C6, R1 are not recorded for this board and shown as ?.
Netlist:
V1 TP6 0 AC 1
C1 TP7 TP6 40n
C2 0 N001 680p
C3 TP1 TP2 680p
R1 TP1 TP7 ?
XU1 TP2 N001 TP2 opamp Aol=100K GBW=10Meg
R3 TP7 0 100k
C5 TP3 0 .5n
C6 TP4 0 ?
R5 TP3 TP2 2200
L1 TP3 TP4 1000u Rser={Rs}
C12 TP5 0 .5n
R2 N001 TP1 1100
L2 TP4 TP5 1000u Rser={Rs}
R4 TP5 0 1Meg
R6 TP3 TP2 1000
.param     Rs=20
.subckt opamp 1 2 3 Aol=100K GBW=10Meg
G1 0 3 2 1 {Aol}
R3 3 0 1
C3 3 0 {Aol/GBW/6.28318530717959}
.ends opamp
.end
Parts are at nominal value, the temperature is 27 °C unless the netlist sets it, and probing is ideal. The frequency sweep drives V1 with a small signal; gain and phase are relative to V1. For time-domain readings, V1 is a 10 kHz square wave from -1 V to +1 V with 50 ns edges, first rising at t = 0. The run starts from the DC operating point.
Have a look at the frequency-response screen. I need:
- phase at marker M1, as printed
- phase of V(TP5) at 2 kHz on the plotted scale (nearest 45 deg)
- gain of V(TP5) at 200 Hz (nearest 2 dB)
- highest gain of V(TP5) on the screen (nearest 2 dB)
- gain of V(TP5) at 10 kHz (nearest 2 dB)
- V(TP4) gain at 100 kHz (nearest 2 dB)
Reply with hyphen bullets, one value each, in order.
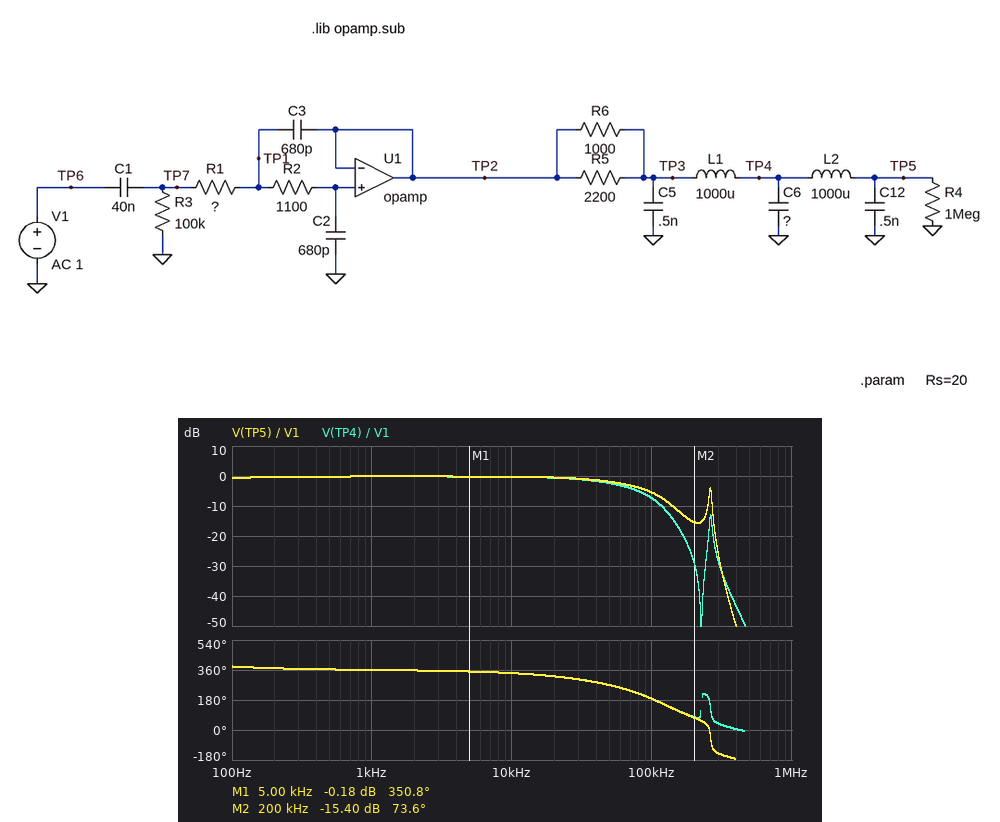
- 350.8 deg
- 360 deg
- 0 dB
- 0 dB
- 0 dB
- -8 dB
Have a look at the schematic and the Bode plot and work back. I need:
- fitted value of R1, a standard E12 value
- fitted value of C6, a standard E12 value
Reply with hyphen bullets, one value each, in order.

- 3.9 kΩ
- 1.8 nF
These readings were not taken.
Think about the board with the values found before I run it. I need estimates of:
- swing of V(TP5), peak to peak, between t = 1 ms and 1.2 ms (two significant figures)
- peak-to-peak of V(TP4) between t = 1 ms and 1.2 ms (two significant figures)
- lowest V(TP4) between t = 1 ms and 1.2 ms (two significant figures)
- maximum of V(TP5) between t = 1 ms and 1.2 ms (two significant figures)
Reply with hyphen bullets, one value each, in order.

- 2.0 V
- 2.0 V
- -260 mV
- 1.8 V
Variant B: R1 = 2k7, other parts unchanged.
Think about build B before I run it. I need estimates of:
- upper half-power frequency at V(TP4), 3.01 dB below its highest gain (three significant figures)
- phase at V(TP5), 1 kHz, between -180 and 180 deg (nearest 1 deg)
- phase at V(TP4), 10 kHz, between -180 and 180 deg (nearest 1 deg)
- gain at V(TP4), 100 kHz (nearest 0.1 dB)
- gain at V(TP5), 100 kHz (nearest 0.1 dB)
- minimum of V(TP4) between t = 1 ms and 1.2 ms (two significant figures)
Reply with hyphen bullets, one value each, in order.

- 78.5 kHz
- 1 deg
- -16 deg
- -5.3 dB
- -3.4 dB
- -270 mV
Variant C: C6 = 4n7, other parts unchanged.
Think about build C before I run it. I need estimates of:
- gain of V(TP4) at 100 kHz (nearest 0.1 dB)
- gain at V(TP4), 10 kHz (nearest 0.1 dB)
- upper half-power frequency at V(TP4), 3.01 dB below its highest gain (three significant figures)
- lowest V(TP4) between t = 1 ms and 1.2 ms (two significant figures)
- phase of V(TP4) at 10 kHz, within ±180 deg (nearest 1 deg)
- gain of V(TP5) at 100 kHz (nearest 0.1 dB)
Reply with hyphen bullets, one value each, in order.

- -14.3 dB
- -0.4 dB
- 38.7 kHz
- -250 mV
- -26 deg
- -12.4 dB
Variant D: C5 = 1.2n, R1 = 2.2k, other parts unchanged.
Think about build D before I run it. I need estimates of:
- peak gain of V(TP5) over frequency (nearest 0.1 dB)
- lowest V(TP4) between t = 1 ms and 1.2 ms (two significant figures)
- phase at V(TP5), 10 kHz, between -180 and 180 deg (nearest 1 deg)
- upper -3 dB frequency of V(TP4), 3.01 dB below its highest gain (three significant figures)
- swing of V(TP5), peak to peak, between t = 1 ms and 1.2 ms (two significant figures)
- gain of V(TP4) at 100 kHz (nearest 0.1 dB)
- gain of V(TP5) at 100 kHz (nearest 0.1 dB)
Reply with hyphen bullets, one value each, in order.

- 0.9 dB
- -270 mV
- -17 deg
- 77.7 kHz
- 2.1 V
- -4.5 dB
- -2.6 dB
